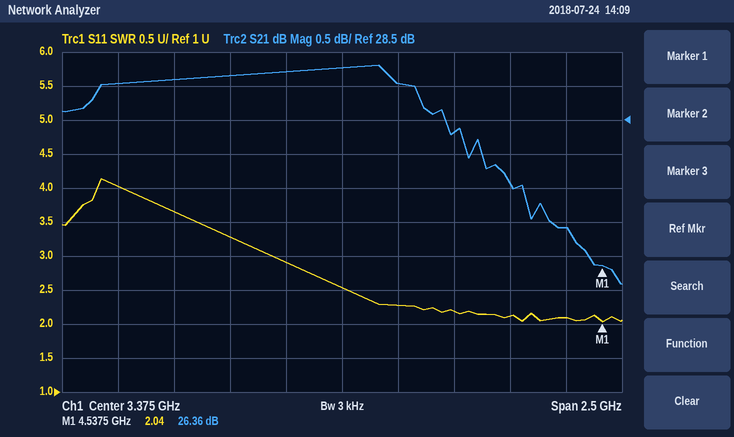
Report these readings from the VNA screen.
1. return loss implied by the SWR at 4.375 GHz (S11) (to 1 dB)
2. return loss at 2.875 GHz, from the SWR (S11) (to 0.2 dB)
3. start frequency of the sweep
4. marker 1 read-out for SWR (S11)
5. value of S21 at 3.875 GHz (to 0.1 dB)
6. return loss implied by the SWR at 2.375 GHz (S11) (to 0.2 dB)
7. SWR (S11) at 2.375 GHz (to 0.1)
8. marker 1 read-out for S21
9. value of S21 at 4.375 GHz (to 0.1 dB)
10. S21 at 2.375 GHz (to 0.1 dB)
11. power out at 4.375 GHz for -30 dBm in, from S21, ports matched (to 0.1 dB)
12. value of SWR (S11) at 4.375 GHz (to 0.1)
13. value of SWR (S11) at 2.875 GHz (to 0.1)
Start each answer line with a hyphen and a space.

- 9 dB
- 5.4 dB
- 2.125 GHz
- 2.04
- 28.3 dB
- 4.4 dB
- 4.0
- 26.36 dB
- 26.9 dB
- 29.0 dB
- -3.1 dBm
- 2.1
- 3.3
